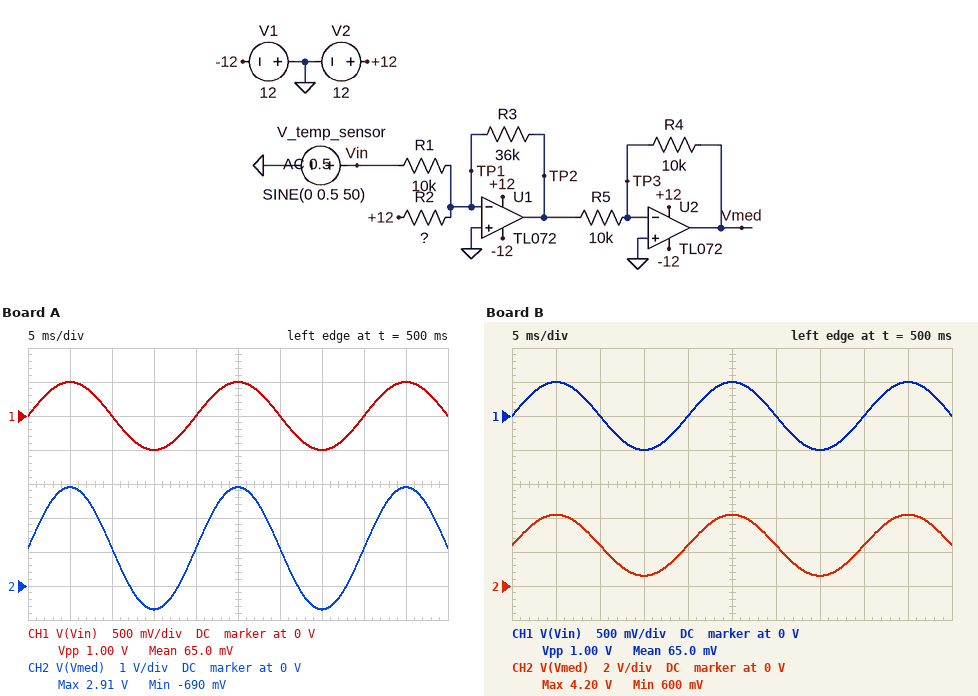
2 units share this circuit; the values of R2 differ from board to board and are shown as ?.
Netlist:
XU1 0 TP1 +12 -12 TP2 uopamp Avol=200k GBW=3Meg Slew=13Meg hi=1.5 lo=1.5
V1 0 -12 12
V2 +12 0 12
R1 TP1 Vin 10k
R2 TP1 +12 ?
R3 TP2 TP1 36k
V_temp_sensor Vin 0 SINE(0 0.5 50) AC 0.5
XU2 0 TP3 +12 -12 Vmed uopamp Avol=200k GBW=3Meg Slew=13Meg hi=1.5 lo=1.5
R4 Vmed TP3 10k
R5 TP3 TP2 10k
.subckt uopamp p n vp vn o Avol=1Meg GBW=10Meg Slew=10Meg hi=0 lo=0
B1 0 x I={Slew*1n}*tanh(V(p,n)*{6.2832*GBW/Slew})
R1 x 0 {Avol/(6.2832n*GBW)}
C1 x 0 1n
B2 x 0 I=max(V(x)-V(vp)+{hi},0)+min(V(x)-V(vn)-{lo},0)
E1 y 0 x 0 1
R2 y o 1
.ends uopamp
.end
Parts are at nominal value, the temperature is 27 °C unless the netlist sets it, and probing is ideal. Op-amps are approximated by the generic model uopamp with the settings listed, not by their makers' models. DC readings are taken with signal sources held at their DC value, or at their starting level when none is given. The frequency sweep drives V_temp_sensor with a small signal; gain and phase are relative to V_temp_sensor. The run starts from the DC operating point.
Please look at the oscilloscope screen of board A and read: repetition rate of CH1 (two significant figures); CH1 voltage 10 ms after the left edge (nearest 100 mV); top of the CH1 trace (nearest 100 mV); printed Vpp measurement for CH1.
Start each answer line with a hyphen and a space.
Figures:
- 50 Hz
- 0 V
- 500 mV
- 1.00 V
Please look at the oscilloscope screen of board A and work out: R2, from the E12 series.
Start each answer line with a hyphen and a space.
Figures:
- 390 kΩ
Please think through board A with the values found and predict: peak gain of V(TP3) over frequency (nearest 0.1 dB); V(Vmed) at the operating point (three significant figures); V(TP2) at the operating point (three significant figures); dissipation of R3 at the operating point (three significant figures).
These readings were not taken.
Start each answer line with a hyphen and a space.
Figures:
- -5.4 dB
- 1.11 V
- -1.11 V
- 34.1 µW
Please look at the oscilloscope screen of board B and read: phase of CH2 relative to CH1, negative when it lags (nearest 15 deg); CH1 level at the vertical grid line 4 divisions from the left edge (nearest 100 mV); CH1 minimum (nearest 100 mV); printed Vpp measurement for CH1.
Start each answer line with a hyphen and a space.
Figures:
- 0 deg
- 0 V
- -500 mV
- 1.00 V
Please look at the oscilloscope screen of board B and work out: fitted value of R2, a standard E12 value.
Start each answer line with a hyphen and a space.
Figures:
- 180 kΩ
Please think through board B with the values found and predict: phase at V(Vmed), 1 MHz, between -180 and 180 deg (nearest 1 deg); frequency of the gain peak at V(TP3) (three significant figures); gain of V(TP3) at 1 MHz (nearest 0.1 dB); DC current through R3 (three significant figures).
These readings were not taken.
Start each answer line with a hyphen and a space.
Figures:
- -92 deg
- 968 kHz
- -5.5 dB
- 66.7 µA
